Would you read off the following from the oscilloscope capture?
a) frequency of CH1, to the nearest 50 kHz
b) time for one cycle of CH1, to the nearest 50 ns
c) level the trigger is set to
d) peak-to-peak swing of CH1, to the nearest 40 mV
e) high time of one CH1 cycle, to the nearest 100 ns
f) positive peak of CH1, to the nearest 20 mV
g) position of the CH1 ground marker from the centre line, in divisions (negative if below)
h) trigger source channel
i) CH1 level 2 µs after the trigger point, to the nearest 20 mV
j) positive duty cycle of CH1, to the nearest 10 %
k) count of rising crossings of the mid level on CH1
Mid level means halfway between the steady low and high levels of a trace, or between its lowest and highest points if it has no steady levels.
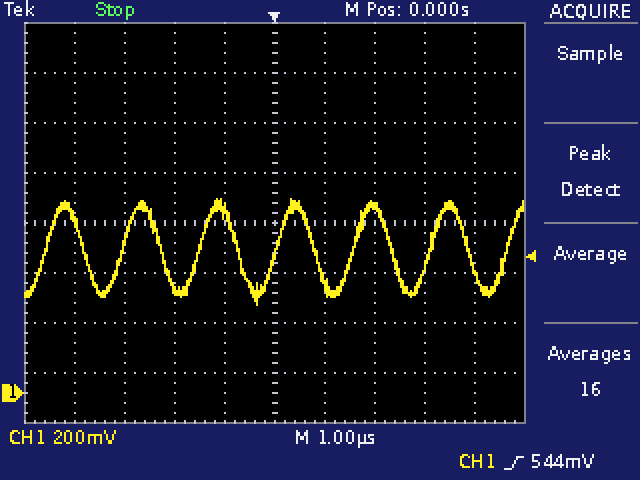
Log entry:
650 kHz
1.55 µs
544 mV
440 mV
800 ns
780 mV
-3.4 div
CH1
740 mV
50 %
7
